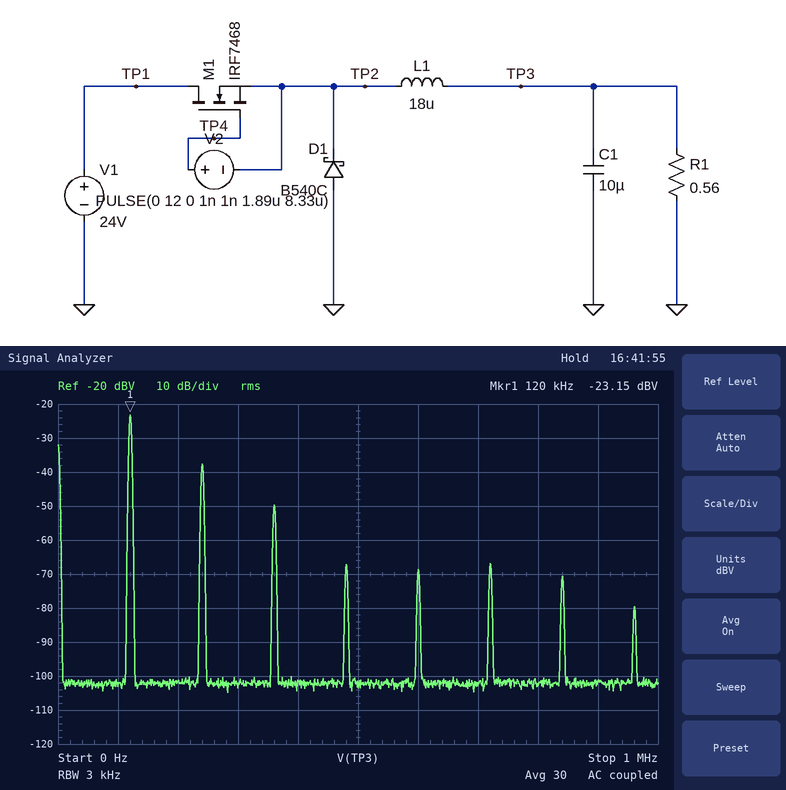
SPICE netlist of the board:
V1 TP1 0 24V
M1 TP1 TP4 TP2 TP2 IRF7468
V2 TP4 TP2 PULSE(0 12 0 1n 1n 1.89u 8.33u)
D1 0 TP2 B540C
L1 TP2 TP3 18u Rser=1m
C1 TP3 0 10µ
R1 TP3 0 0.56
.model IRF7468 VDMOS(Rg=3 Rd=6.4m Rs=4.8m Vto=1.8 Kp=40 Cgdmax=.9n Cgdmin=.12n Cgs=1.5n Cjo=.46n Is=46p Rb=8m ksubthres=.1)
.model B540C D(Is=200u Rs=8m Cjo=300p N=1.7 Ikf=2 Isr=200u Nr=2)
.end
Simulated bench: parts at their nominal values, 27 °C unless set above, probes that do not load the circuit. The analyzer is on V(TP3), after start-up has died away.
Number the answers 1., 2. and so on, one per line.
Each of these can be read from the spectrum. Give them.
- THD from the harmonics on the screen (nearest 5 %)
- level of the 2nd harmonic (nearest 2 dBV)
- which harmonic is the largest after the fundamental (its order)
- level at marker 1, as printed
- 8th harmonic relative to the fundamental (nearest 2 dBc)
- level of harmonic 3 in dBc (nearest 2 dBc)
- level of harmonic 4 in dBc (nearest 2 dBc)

1. 20 %
2. -38 dBV
3. 2
4. -23.15 dBV
5. -56 dBc
6. -26 dBc
7. -44 dBc
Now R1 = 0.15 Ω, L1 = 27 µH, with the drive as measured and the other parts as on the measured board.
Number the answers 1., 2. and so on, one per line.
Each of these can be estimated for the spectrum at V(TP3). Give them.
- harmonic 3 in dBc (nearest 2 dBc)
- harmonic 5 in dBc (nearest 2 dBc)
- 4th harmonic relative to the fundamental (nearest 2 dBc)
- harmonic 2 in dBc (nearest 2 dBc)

1. -24 dBc
2. -44 dBc
3. -42 dBc
4. -12 dBc
